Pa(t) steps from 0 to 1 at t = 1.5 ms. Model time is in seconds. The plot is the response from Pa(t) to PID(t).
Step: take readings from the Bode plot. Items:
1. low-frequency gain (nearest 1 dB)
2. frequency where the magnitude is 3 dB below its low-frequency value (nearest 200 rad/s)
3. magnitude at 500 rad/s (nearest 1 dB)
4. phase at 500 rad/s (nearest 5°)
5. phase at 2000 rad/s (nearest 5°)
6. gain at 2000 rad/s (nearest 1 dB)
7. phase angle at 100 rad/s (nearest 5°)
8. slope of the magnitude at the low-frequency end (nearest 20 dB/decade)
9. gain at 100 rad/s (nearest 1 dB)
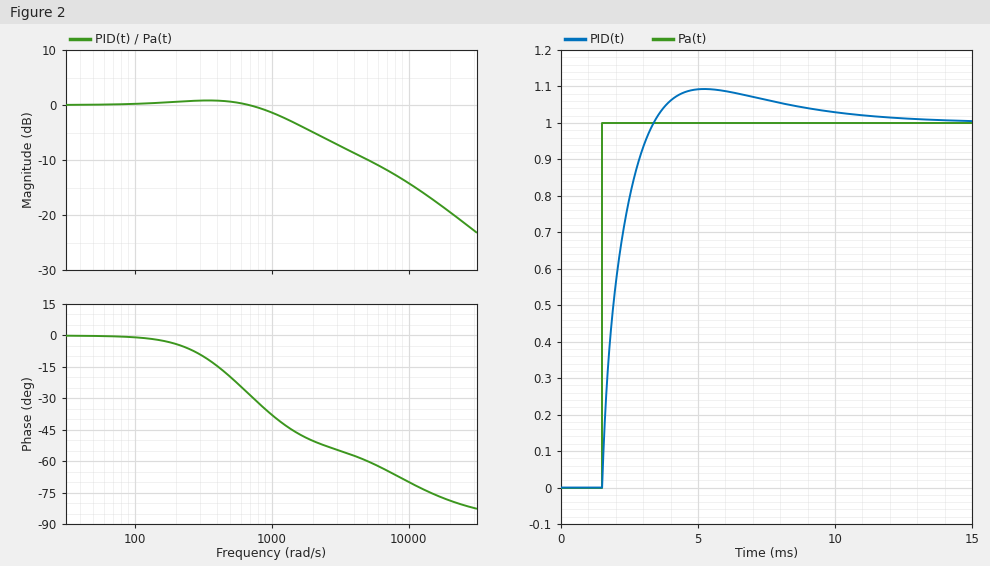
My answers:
0 dB
1400 rad/s
1 dB
-20°
-50°
-5 dB
0°
0 dB/decade
0 dB
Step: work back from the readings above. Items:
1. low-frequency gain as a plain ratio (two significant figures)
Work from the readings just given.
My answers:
1.0
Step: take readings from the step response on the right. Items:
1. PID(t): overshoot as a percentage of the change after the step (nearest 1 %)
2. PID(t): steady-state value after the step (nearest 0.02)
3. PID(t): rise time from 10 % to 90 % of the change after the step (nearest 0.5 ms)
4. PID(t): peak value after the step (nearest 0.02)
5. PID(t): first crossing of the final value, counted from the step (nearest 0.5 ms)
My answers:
9 %
1.00
1.5 ms
1.10
2.0 ms
